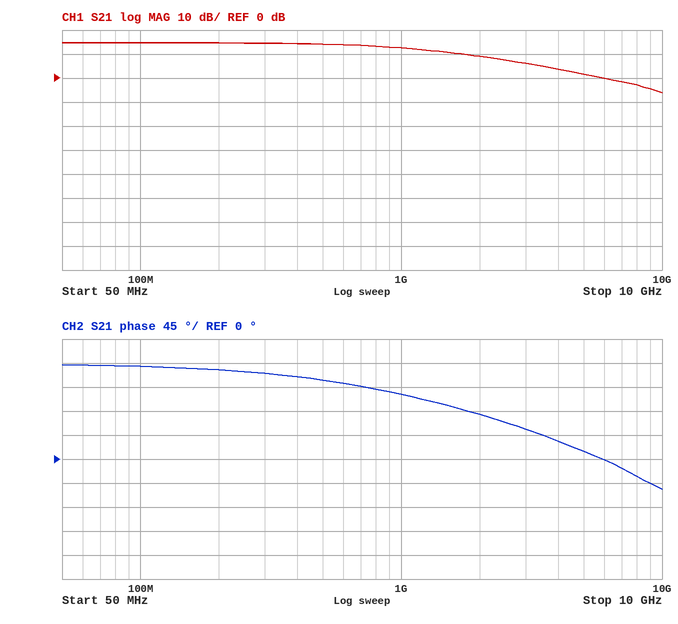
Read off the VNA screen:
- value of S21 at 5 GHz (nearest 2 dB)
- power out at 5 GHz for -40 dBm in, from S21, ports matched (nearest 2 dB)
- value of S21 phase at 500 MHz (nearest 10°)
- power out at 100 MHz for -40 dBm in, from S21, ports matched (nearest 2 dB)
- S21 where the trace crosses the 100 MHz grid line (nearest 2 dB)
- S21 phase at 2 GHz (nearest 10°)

2 dB
-38 dBm
150°
-26 dBm
14 dB
80°
